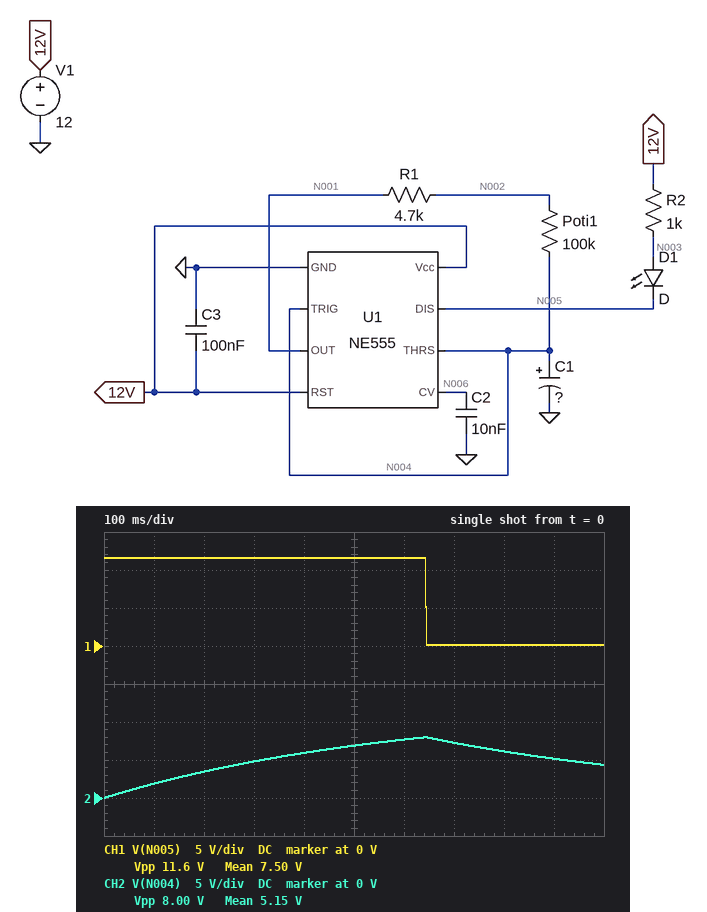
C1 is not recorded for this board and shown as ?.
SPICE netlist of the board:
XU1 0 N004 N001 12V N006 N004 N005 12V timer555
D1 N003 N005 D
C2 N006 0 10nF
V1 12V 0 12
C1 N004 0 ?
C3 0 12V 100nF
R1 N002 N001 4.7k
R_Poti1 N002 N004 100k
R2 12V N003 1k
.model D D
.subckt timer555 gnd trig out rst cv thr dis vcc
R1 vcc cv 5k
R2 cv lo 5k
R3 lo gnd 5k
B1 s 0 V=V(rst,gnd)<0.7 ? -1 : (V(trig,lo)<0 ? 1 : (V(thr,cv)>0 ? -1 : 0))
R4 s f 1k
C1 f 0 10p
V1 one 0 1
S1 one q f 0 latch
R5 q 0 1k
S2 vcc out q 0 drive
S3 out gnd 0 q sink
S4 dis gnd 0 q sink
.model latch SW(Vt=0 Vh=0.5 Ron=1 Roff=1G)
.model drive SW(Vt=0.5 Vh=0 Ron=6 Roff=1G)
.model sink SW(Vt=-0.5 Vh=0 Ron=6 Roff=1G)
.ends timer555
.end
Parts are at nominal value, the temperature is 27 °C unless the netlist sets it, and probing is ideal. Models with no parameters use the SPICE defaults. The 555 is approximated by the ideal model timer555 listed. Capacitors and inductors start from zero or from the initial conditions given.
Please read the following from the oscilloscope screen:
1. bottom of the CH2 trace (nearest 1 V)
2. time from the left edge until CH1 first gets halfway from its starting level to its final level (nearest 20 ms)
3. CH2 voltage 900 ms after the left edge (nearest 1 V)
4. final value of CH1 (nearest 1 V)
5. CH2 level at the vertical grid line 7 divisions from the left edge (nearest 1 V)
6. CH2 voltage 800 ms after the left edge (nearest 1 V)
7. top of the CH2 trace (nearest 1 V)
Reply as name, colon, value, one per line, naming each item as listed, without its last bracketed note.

bottom of the CH2 trace: 0 V
time from the left edge until CH1 first gets halfway from its starting level to its final level: 640 ms
CH2 voltage 900 ms after the left edge: 5 V
final value of CH1: 0 V
CH2 level at the vertical grid line 7 divisions from the left edge: 7 V
CH2 voltage 800 ms after the left edge: 6 V
top of the CH2 trace: 8 V
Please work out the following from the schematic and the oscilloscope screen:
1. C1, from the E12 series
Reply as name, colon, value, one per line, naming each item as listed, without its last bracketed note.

C1, from the E12 series: 5.6 µF
